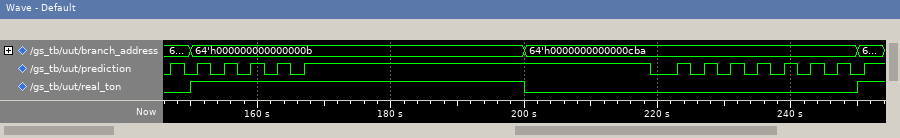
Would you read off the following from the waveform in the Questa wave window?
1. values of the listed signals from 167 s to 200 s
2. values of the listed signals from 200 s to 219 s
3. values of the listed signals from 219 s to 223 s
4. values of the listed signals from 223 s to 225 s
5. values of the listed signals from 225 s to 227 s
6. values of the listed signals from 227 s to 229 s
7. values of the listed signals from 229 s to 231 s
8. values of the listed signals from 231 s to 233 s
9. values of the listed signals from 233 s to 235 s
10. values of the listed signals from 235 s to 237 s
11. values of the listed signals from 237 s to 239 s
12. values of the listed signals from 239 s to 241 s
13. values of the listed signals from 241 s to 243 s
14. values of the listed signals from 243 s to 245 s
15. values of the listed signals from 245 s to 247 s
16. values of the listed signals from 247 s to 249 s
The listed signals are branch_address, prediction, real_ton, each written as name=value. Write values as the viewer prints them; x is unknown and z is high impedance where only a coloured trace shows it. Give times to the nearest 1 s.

branch_address=64'h000000000000000b, prediction=1, real_ton=1
branch_address=64'h0000000000000cba, prediction=1, real_ton=0
branch_address=64'h0000000000000cba, prediction=0, real_ton=0
branch_address=64'h0000000000000cba, prediction=1, real_ton=0
branch_address=64'h0000000000000cba, prediction=0, real_ton=0
branch_address=64'h0000000000000cba, prediction=1, real_ton=0
branch_address=64'h0000000000000cba, prediction=0, real_ton=0
branch_address=64'h0000000000000cba, prediction=1, real_ton=0
branch_address=64'h0000000000000cba, prediction=0, real_ton=0
branch_address=64'h0000000000000cba, prediction=1, real_ton=0
branch_address=64'h0000000000000cba, prediction=0, real_ton=0
branch_address=64'h0000000000000cba, prediction=1, real_ton=0
branch_address=64'h0000000000000cba, prediction=0, real_ton=0
branch_address=64'h0000000000000cba, prediction=1, real_ton=0
branch_address=64'h0000000000000cba, prediction=0, real_ton=0
branch_address=64'h0000000000000cba, prediction=1, real_ton=0
